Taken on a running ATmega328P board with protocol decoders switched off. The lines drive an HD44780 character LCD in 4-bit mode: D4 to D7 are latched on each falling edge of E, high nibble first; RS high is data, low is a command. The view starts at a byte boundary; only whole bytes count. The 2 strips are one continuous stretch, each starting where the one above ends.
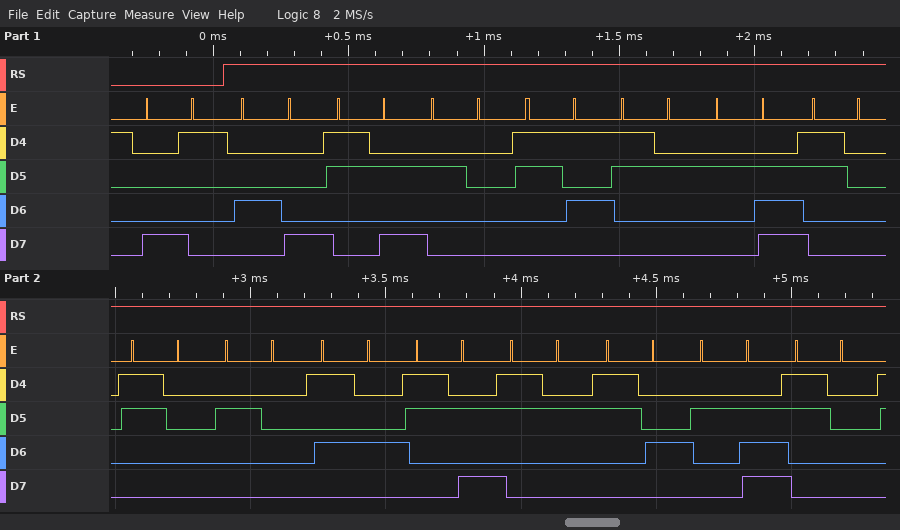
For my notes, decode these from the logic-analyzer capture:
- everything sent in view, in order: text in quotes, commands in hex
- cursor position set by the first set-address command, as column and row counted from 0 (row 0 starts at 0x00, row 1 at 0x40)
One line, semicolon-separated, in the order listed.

0x81 "H: 52.00 T:24.0"; column 1, row 0
